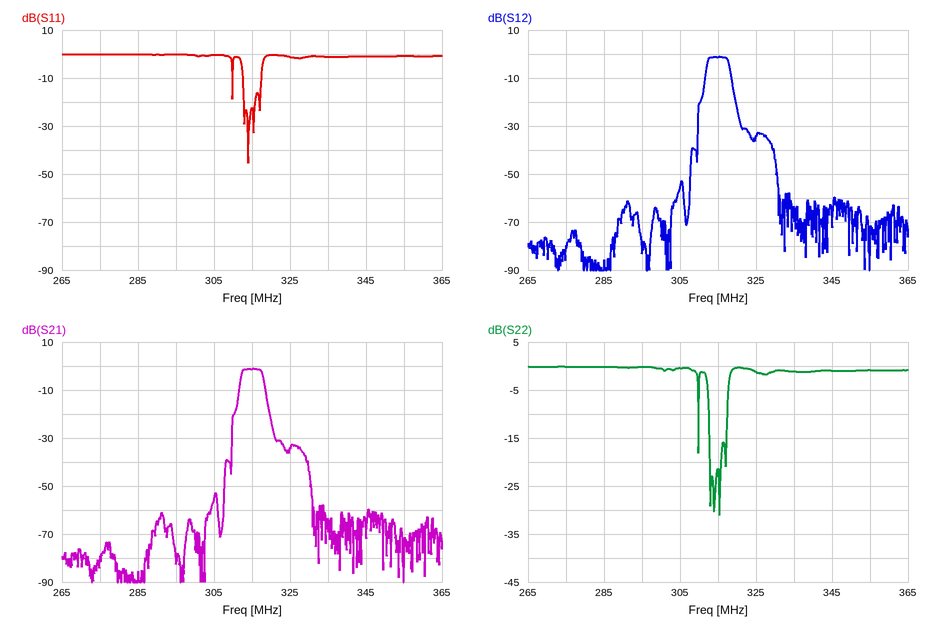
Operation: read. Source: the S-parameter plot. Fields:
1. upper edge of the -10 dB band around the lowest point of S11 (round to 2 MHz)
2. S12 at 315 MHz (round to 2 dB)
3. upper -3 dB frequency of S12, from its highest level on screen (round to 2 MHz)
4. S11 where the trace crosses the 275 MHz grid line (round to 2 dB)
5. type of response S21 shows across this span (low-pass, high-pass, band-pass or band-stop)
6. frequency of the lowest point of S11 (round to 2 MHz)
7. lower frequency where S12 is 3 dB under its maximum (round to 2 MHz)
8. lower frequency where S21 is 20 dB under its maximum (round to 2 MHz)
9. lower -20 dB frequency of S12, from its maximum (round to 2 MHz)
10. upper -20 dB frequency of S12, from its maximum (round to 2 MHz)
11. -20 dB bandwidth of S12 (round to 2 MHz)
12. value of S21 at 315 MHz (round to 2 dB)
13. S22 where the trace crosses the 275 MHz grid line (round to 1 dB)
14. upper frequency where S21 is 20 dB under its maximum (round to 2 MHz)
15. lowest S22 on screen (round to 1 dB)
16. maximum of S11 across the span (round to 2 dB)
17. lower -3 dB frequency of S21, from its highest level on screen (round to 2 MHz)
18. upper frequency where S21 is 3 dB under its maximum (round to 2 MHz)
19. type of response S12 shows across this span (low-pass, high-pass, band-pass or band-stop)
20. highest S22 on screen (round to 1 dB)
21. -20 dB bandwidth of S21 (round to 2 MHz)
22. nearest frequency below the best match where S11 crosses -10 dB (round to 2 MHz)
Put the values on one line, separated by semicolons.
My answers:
318 MHz; -2 dB; 318 MHz; 0 dB; band-pass; 314 MHz; 312 MHz; 310 MHz; 310 MHz; 320 MHz; 10 MHz; -2 dB; 0 dB; 320 MHz; -31 dB; 0 dB; 312 MHz; 318 MHz; band-pass; 0 dB; 10 MHz; 312 MHz
